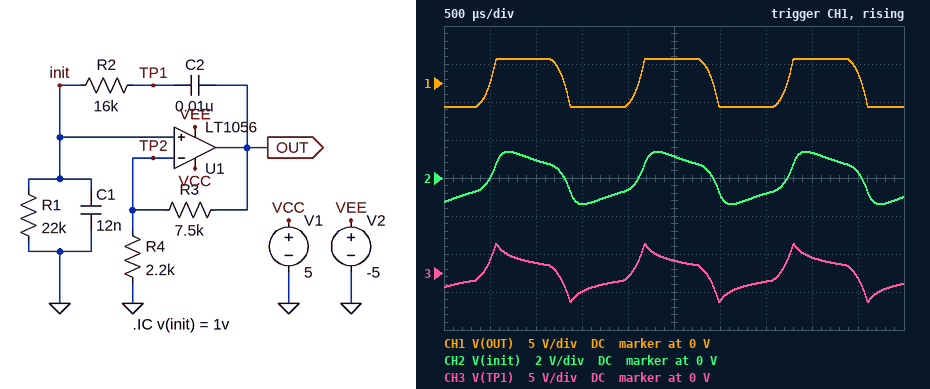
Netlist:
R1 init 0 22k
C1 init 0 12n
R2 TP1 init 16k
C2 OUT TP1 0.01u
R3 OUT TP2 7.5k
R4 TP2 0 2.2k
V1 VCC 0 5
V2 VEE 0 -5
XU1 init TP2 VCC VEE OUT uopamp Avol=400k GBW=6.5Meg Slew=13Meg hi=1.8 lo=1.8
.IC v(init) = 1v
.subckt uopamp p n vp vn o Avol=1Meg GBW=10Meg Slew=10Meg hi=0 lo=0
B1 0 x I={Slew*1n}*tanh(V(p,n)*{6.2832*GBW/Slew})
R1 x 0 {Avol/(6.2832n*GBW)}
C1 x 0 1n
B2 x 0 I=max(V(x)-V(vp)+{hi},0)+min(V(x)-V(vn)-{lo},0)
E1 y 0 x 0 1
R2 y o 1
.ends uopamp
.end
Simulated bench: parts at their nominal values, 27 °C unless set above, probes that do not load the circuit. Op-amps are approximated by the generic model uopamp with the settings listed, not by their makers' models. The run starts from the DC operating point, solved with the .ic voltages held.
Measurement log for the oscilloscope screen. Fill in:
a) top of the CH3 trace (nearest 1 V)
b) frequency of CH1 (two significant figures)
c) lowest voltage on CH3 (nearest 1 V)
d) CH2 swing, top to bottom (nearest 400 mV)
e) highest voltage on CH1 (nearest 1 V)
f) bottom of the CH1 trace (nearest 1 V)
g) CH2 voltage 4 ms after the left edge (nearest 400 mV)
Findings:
4 V
620 Hz
-4 V
2.8 V
3 V
-3 V
1.2 V
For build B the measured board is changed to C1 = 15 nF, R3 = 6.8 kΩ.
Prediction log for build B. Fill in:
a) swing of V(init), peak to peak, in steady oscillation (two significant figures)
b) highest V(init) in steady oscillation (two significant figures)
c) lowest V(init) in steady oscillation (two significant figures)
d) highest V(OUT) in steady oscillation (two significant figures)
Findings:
2.4 V
1.2 V
-1.2 V
3.2 V
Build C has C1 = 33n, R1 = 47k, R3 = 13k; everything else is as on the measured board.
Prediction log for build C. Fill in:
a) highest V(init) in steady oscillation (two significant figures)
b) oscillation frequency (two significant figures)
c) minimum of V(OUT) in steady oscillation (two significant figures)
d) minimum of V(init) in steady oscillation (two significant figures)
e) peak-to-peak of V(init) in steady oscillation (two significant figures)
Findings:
880 mV
220 Hz
-3.2 V
-880 mV
1.8 V
